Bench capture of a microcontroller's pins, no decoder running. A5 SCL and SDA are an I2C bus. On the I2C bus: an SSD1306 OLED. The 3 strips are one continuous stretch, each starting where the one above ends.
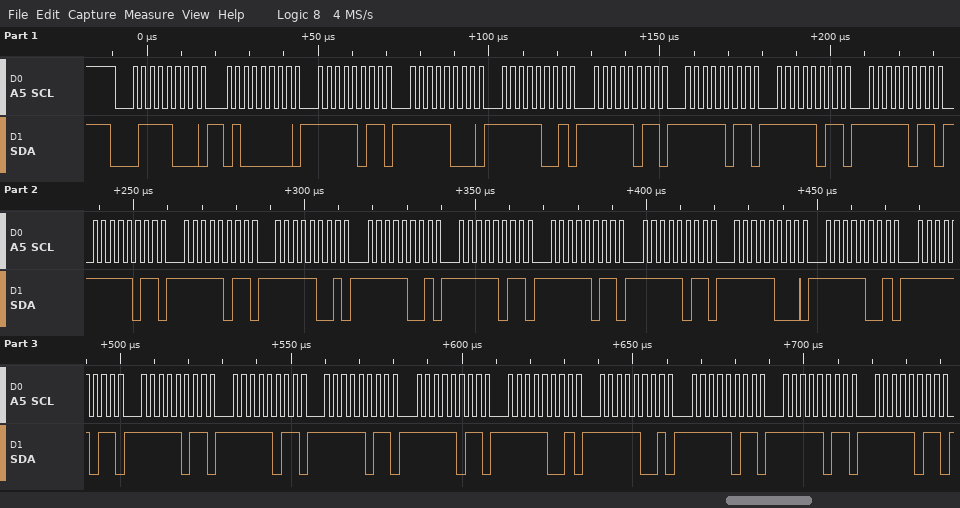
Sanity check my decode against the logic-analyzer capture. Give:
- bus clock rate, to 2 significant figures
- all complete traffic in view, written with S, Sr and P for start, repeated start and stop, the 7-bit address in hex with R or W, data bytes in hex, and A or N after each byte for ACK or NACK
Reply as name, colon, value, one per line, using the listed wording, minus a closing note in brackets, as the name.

bus clock rate, to 2 significant figures: 400 kHz
all complete traffic in view, written with S, Sr and P for start, repeated start and stop, the 7-bit address in hex with R or W, data bytes in hex, and A or N after each byte for ACK or NACK: S 3CW A 40 A FB A F8 A F9 A FB A FB A FB A FB A FB A FB A F9 A F9 A FB A FB A FB A F8 A F9 A FB A FB A FB A FB A FB A F9 A F9 A FB A FB A FB A
